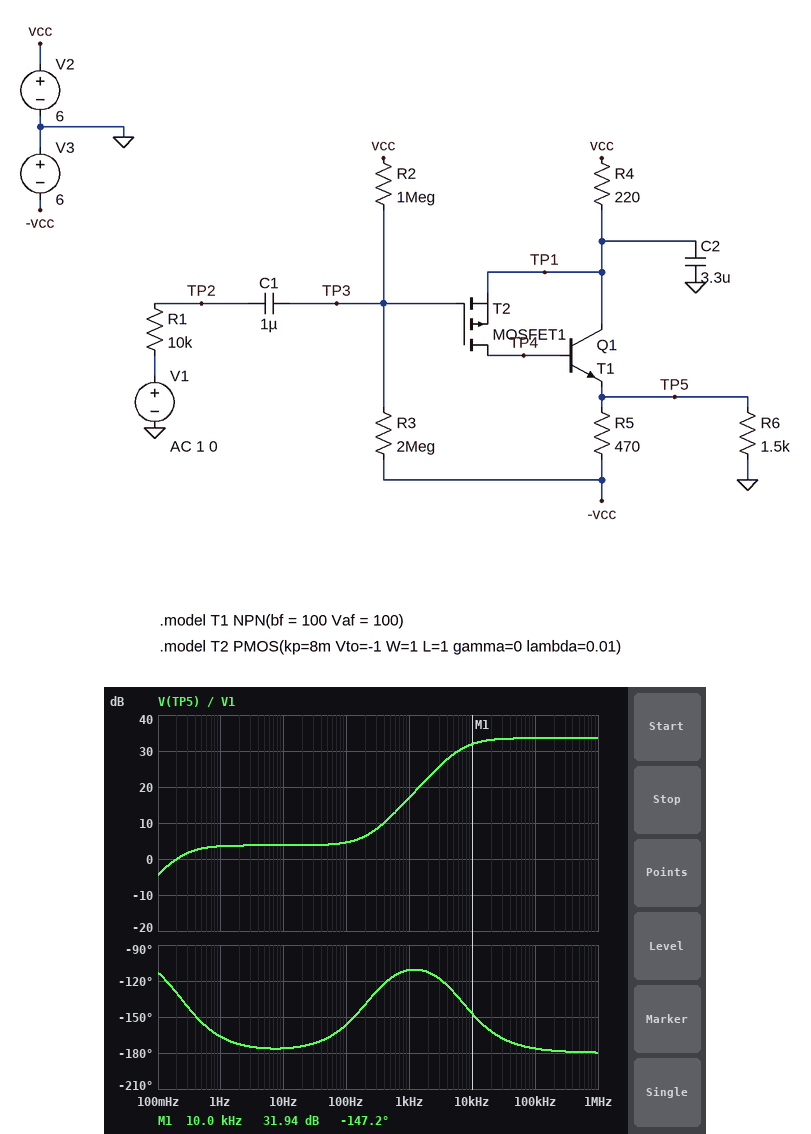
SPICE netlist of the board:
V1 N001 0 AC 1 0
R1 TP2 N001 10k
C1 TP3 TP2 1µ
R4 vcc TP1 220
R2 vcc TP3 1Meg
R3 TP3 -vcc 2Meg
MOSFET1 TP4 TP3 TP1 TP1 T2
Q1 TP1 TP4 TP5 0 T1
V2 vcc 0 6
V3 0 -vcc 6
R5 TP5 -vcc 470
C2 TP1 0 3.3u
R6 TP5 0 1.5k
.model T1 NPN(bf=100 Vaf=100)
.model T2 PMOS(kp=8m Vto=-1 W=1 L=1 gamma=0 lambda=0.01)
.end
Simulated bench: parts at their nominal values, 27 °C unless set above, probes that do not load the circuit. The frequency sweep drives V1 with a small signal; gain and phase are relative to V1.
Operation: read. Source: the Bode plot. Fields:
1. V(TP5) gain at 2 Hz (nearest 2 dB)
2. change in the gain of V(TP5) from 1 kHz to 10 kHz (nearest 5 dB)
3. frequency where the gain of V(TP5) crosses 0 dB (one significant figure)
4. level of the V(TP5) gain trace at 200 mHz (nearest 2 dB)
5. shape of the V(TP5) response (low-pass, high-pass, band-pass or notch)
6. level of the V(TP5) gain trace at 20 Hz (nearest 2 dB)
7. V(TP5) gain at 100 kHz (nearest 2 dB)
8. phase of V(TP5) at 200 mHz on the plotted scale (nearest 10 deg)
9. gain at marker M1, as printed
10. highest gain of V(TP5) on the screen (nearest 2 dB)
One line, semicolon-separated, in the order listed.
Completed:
4 dB; 15 dB; 200 mHz; 0 dB; high-pass; 4 dB; 34 dB; -130 deg; 31.94 dB; 34 dB
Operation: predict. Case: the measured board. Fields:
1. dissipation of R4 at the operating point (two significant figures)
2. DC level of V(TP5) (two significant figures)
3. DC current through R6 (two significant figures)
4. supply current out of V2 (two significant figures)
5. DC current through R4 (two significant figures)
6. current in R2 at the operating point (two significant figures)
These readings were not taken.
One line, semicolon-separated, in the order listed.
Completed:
36 mW; 28 mV; 19 µA; 13 mA; 13 mA; 4.0 µA
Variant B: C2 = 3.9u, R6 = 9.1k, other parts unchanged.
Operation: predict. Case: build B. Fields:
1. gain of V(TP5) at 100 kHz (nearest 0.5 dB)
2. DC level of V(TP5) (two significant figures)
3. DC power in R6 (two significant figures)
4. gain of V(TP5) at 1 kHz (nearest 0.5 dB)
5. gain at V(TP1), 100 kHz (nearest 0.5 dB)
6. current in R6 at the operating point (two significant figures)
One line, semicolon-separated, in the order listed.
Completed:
35.5 dB; 35 mV; 130 nW; 20.5 dB; -25.5 dB; 3.8 µA
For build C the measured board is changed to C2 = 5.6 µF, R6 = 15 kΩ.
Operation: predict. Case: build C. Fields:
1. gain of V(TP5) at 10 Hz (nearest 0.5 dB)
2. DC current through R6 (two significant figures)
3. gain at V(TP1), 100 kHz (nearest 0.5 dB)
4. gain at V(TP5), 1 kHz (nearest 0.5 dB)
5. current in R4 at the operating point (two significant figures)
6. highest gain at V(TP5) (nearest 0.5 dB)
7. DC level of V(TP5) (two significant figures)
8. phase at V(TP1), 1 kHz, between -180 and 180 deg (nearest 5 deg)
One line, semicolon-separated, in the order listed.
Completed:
6.0 dB; 2.4 µA; -28.5 dB; 23.5 dB; 13 mA; 35.5 dB; 36 mV; -15 deg
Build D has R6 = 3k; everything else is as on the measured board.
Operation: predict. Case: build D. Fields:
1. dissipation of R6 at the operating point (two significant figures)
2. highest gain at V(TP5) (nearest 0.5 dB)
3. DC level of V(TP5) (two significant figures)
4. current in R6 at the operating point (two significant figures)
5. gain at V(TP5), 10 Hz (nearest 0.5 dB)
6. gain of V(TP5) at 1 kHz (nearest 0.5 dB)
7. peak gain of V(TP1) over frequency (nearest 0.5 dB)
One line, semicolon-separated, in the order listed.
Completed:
340 nW; 34.5 dB; 32 mV; 11 µA; 5.0 dB; 18.0 dB; -0.5 dB
